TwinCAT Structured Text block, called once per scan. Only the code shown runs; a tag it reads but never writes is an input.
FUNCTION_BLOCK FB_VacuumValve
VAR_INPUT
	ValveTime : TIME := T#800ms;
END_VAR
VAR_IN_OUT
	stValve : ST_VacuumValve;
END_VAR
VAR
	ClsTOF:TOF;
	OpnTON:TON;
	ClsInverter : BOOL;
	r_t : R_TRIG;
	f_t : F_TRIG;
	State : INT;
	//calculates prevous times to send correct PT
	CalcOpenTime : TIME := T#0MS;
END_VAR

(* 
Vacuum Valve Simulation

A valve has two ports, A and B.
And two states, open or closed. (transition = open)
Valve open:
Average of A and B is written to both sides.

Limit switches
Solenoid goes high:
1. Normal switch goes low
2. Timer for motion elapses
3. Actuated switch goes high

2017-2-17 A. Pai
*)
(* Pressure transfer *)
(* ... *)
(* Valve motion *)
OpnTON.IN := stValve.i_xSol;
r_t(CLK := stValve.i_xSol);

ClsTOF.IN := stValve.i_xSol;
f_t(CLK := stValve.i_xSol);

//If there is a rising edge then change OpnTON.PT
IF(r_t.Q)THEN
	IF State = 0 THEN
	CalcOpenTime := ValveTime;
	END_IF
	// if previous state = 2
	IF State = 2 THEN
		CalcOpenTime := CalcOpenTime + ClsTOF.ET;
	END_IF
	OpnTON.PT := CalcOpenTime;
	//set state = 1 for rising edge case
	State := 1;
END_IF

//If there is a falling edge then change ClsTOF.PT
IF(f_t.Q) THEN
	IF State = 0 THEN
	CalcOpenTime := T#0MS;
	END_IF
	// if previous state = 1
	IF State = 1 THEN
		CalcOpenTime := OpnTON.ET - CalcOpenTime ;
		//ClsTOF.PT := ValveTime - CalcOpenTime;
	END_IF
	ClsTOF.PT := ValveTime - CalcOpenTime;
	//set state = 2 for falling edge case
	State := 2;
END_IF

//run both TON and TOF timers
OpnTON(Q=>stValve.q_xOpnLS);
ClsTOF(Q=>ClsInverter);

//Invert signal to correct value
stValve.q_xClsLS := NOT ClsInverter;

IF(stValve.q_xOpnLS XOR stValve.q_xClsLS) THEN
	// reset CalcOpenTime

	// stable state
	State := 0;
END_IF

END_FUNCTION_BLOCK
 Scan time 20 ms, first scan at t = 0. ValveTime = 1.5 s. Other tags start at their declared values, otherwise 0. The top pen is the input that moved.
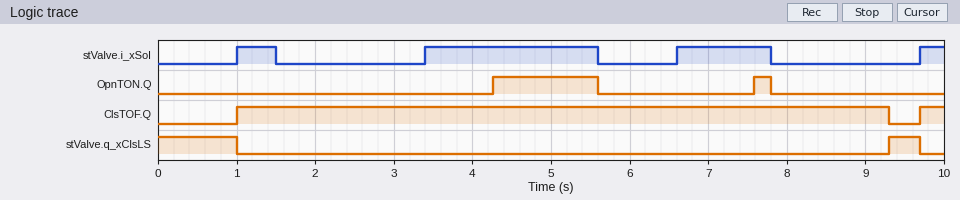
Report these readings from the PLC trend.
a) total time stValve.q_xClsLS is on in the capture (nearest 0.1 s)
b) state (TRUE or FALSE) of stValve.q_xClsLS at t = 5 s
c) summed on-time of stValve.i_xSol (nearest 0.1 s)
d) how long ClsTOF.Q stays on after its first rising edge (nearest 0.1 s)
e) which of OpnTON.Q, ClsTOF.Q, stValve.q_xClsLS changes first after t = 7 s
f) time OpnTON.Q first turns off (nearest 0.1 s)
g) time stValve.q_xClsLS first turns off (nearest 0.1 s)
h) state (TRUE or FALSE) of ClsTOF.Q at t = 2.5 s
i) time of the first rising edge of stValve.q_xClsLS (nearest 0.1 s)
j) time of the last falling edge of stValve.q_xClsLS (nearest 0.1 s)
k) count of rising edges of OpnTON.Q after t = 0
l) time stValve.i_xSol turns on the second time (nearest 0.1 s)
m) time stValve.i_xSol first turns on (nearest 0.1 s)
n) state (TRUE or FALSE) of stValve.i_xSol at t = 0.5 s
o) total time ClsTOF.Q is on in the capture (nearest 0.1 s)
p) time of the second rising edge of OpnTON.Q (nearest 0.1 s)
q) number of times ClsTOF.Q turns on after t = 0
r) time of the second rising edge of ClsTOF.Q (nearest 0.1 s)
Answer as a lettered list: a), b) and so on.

a) 1.4 s
b) FALSE
c) 4.2 s
d) 8.3 s
e) OpnTON.Q
f) 5.6 s
g) 1.0 s
h) TRUE
i) 9.3 s
j) 9.7 s
k) 2
l) 3.4 s
m) 1.0 s
n) FALSE
o) 8.6 s
p) 7.6 s
q) 2
r) 9.7 s
